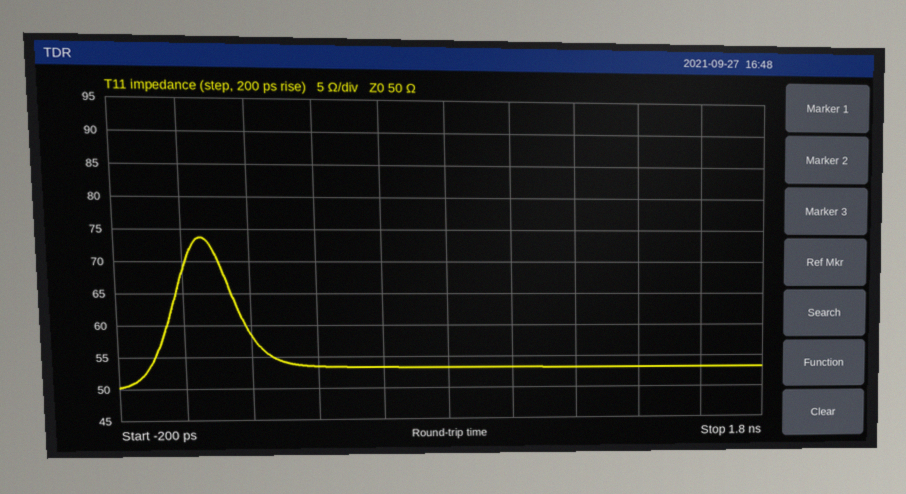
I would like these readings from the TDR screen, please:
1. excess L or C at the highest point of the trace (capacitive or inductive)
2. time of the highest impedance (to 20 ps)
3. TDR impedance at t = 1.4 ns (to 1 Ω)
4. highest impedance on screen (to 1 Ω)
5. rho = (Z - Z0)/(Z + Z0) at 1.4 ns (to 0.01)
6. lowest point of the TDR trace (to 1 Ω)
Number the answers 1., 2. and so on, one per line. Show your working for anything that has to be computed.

1. inductive
2. 60 ps
3. 53 Ω
4. 74 Ω
5. (53 − 50)/(53 + 50) ≈ +0.03
6. 50 Ω
